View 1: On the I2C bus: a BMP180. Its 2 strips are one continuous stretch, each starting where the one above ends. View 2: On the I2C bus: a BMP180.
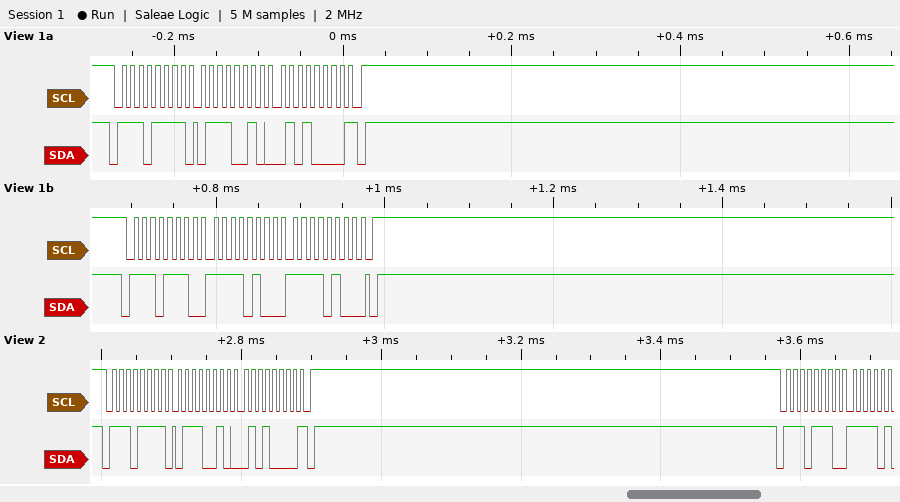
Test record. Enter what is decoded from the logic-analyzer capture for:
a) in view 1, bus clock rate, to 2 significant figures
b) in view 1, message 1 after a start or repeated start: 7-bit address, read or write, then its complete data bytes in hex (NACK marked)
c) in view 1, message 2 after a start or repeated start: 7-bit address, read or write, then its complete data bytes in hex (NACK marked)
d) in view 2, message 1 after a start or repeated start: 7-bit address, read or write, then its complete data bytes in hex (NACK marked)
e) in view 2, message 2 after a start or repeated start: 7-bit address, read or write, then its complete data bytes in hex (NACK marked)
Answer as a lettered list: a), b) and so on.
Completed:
a) 100 kHz
b) 0x77 read: 72 50 NACK
c) 0x77 write: F4 F4
d) 0x77 read: 72 50 NACK
e) 0x77 write
